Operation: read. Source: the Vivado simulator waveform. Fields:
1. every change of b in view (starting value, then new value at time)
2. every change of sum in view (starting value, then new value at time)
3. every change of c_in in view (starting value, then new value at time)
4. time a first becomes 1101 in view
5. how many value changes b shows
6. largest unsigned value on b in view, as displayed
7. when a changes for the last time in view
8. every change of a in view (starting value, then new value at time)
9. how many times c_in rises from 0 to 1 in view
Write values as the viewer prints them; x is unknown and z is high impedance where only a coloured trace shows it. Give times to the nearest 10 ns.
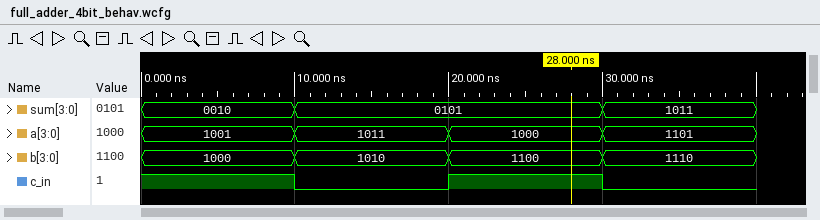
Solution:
1000, 1010 at 10 ns, 1100 at 20 ns, 1110 at 30 ns
0010, 0101 at 10 ns, 1011 at 30 ns
1, 0 at 10 ns, 1 at 20 ns, 0 at 30 ns
30 ns
3
1110
30 ns
1001, 1011 at 10 ns, 1000 at 20 ns, 1101 at 30 ns
1
